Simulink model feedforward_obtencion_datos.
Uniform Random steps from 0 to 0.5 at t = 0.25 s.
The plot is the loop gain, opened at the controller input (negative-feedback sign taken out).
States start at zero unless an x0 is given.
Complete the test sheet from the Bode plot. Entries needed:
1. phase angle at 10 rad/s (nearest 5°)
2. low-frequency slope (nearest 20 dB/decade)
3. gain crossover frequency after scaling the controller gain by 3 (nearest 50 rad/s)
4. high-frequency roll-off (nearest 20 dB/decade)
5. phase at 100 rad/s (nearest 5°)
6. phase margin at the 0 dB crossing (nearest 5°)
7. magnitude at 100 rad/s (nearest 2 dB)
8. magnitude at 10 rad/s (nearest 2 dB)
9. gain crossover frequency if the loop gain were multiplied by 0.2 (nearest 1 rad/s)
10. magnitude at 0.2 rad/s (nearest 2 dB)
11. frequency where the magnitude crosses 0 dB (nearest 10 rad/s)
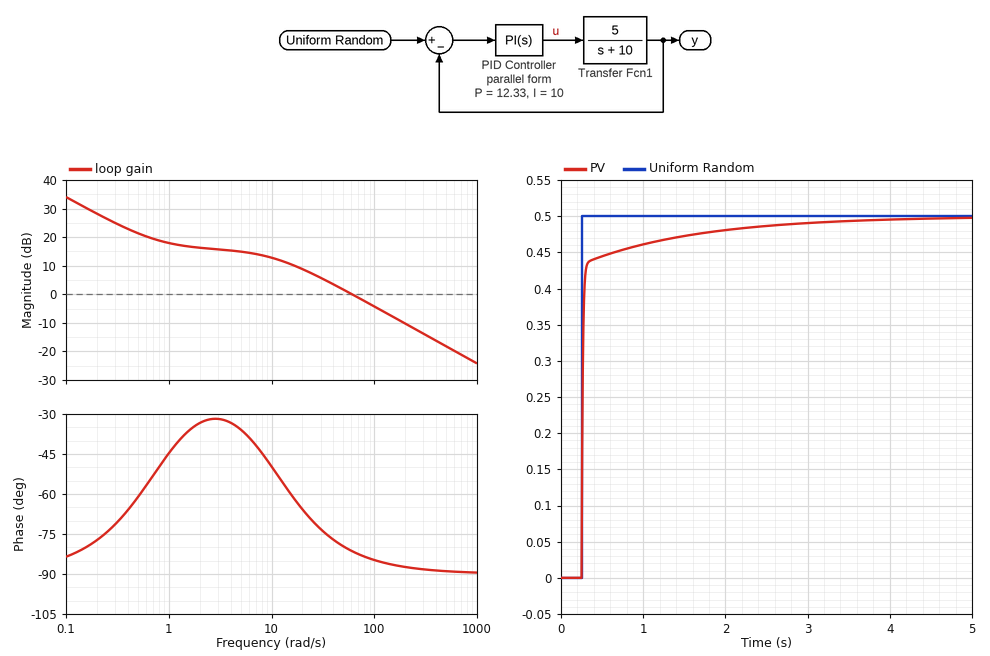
-50°
-20 dB/decade
200 rad/s
-20 dB/decade
-85°
100°
-4 dB
12 dB
7 rad/s
28 dB
60 rad/s
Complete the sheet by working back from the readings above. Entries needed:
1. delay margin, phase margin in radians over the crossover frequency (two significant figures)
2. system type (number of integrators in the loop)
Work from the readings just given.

0.029 s
1
